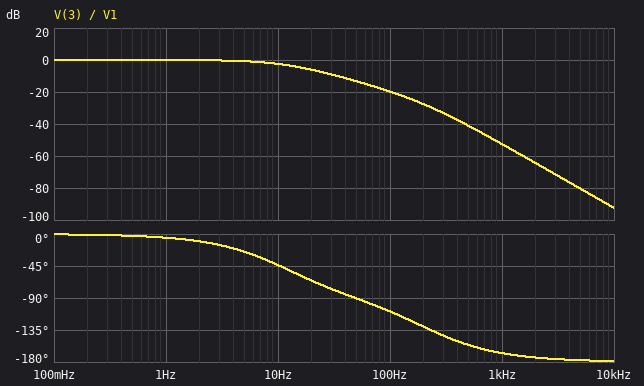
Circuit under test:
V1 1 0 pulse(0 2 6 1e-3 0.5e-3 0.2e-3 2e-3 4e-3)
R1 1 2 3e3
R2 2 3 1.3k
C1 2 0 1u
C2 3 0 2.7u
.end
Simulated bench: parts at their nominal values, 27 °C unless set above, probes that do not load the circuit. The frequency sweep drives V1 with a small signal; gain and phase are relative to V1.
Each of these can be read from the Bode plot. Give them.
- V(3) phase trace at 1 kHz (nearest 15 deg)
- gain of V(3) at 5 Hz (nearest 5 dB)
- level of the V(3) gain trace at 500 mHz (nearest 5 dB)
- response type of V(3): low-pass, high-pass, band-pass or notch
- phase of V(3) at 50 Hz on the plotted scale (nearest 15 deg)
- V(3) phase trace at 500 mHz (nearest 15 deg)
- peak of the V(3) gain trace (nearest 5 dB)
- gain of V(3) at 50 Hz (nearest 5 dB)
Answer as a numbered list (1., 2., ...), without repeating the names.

1. -165 deg
2. 0 dB
3. 0 dB
4. low-pass
5. -90 deg
6. 0 deg
7. 0 dB
8. -15 dB
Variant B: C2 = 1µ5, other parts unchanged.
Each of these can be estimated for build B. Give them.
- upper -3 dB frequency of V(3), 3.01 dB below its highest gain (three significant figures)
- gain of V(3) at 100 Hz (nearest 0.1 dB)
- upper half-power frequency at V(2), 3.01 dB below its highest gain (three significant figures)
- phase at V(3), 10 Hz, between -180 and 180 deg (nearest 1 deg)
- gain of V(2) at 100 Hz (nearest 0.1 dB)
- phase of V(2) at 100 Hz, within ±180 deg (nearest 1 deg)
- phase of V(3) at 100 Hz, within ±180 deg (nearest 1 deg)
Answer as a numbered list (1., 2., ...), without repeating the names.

1. 18.0 Hz
2. -15.7 dB
3. 19.0 Hz
4. -31 deg
5. -11.7 dB
6. -52 deg
7. -102 deg
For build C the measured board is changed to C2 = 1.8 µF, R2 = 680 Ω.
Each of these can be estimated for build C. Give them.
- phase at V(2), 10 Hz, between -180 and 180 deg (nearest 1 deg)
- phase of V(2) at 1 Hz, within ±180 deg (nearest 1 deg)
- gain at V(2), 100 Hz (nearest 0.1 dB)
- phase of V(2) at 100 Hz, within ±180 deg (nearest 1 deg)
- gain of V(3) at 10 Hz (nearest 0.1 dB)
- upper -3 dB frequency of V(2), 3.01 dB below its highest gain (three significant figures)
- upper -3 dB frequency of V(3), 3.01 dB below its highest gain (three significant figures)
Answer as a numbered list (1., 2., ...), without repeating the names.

1. -27 deg
2. -3 deg
3. -13.6 dB
4. -57 deg
5. -1.3 dB
6. 17.5 Hz
7. 17.2 Hz
